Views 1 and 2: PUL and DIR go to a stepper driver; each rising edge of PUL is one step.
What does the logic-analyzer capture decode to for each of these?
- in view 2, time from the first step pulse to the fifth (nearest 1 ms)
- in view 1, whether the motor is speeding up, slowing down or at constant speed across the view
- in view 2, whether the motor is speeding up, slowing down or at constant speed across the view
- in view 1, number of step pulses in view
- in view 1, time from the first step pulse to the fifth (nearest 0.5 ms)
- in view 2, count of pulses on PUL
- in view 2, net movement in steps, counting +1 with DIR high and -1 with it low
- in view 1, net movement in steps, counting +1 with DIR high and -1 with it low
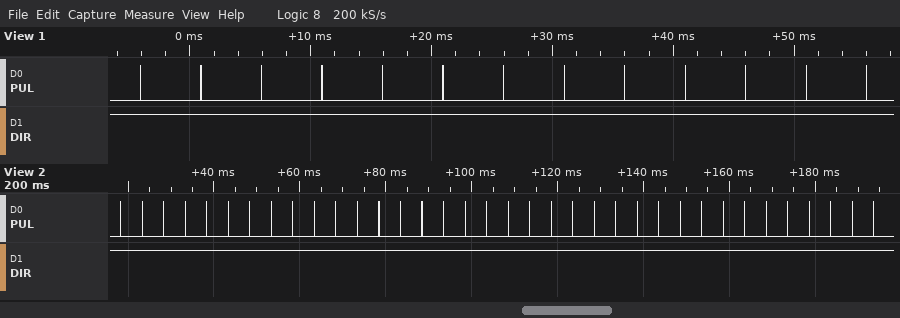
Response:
20 ms
constant speed
constant speed
13
20.0 ms
36
+36
+13
